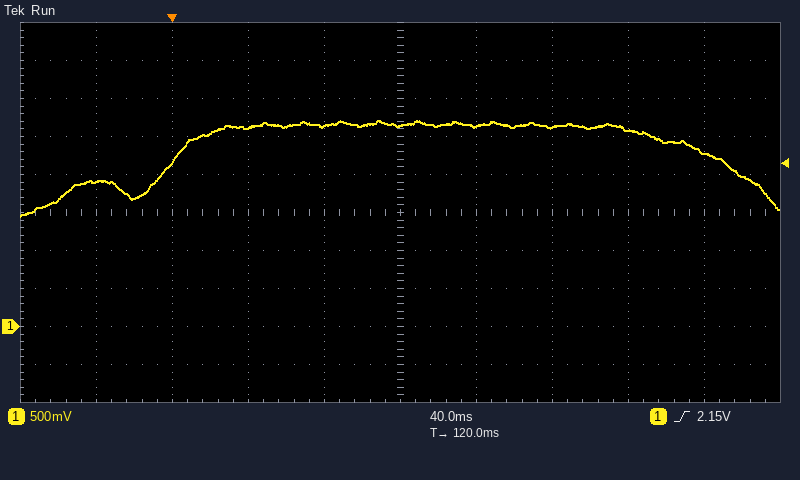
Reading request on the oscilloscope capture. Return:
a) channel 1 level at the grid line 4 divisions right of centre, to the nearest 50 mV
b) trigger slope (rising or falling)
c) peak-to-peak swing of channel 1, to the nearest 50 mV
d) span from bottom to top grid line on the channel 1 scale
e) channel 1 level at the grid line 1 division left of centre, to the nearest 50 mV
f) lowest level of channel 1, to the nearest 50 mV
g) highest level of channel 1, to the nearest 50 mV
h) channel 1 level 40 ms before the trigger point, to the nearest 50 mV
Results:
2.30 V
rising
1.25 V
5 V
2.65 V
1.45 V
2.70 V
1.90 V
